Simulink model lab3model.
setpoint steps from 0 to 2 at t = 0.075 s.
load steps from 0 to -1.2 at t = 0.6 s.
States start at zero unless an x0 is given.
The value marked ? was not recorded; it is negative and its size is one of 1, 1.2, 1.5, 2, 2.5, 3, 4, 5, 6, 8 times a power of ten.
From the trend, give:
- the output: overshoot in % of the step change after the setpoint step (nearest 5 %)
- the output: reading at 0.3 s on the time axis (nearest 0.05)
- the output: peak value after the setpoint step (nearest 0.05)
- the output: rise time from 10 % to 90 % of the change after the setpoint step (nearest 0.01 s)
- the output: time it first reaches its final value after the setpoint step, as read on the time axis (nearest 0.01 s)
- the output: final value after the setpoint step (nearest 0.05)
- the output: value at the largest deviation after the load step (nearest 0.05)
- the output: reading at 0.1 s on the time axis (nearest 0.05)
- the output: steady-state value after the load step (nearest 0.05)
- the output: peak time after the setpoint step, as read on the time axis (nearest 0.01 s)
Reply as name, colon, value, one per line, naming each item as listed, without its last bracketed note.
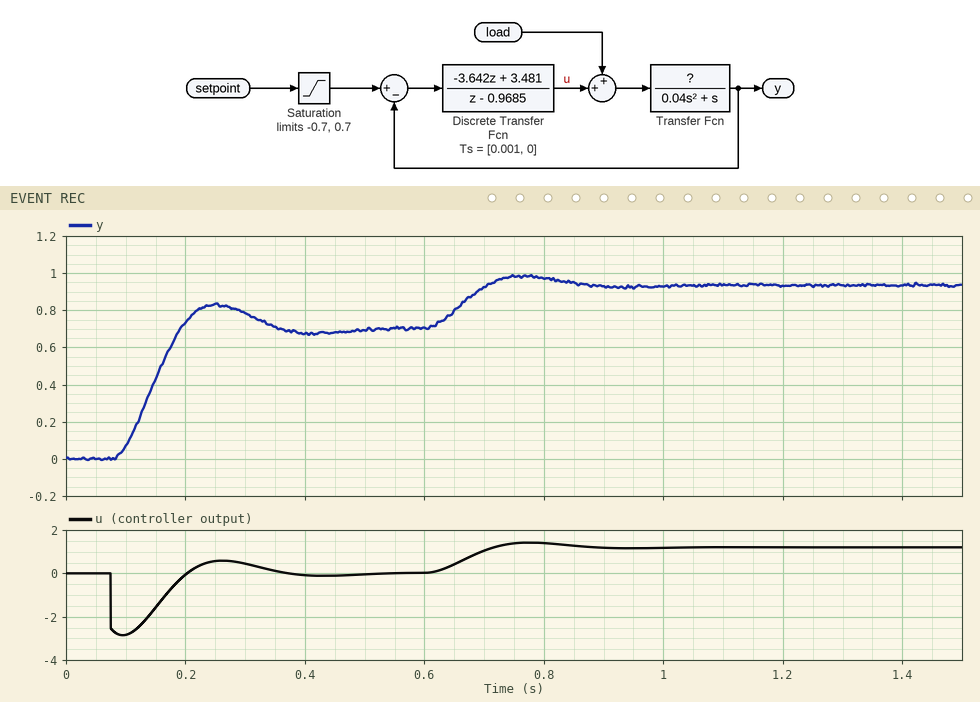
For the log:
the output: overshoot in % of the step change after the setpoint step: 20 %
the output: reading at 0.3 s on the time axis: 0.80
the output: peak value after the setpoint step: 0.85
the output: rise time from 10 % to 90 % of the change after the setpoint step: 0.08 s
the output: time it first reaches its final value after the setpoint step, as read on the time axis: 0.19 s
the output: final value after the setpoint step: 0.70
the output: value at the largest deviation after the load step: 1.00
the output: reading at 0.1 s on the time axis: 0.05
the output: steady-state value after the load step: 0.95
the output: peak time after the setpoint step, as read on the time axis: 0.25 s
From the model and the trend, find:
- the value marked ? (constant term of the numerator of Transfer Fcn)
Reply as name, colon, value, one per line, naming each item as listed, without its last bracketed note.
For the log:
the value marked ?: -4
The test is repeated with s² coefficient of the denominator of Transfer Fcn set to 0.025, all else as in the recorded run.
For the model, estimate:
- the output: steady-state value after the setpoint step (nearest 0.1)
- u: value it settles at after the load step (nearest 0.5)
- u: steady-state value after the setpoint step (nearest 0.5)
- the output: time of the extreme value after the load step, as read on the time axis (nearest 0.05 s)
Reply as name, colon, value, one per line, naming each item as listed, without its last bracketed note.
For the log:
the output: steady-state value after the setpoint step: 0.7
u: value it settles at after the load step: 1.0
u: steady-state value after the setpoint step: 0.0
the output: time of the extreme value after the load step, as read on the time axis: 0.75 s
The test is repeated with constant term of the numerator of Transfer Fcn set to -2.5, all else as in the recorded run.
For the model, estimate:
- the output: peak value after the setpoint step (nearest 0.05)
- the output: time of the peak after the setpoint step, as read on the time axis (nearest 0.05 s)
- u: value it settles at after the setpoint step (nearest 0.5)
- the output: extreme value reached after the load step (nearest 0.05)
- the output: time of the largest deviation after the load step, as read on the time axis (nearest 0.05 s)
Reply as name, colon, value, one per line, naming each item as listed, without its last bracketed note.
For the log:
the output: peak value after the setpoint step: 0.75
the output: time of the peak after the setpoint step, as read on the time axis: 0.30 s
u: value it settles at after the setpoint step: 0.0
the output: extreme value reached after the load step: 0.95
the output: time of the largest deviation after the load step, as read on the time axis: 0.85 s
